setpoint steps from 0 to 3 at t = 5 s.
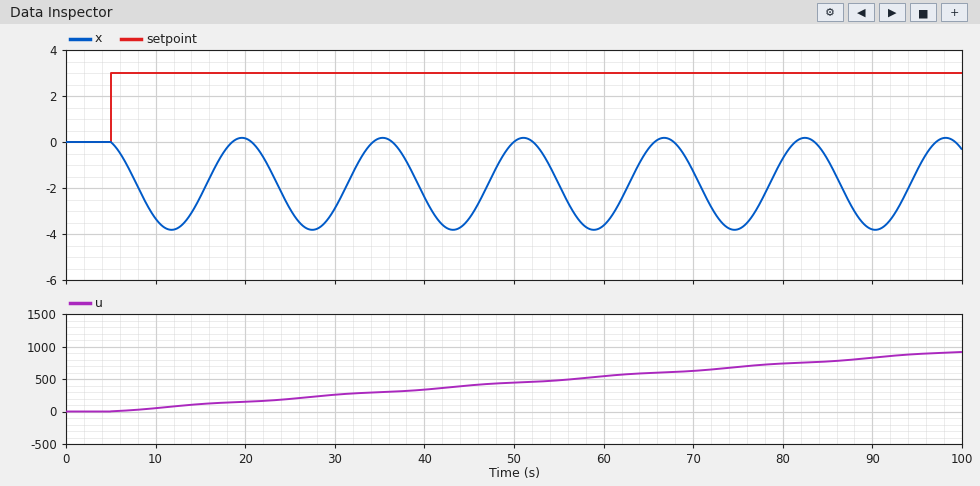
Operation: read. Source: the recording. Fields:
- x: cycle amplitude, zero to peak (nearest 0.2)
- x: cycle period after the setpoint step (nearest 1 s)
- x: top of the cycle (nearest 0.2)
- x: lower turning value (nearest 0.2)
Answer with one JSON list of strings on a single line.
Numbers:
["2.0", "16 s", "0.2", "-3.8"]
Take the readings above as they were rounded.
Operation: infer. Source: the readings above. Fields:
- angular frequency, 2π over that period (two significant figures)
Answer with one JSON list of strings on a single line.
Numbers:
["0.39 rad/s"]
